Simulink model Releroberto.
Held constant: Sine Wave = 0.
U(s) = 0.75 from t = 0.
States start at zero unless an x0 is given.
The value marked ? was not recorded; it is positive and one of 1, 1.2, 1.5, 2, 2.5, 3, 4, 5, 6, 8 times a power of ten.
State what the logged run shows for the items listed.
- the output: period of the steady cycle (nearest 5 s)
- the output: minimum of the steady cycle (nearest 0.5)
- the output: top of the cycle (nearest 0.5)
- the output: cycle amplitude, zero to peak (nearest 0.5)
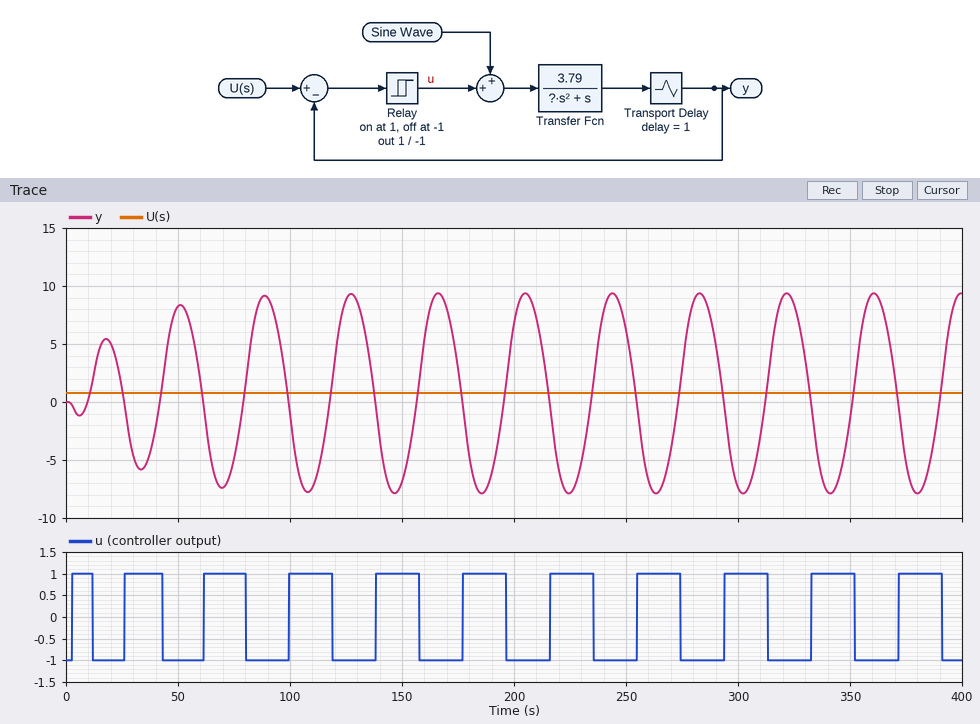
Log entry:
40 s
-8.0
9.5
8.5
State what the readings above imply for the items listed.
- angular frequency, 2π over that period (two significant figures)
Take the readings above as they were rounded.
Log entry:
0.16 rad/s
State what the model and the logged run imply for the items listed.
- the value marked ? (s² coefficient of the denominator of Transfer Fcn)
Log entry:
20
